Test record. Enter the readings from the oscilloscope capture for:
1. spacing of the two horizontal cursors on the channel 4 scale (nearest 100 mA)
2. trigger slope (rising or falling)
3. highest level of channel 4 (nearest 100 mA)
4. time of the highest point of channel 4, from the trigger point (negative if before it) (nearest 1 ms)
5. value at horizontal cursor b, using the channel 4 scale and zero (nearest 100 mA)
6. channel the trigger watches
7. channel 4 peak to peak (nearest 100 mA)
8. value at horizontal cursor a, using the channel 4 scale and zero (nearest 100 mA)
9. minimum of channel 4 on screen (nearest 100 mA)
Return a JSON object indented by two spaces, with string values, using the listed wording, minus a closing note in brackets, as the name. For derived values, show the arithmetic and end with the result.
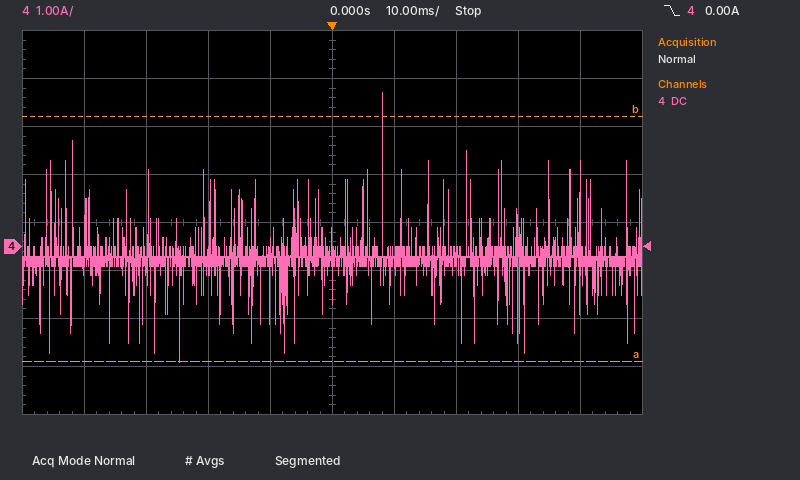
{
  "spacing of the two horizontal cursors on the channel 4 scale": "5.1 A",
  "trigger slope": "falling",
  "highest level of channel 4": "3.2 A",
  "time of the highest point of channel 4, from the trigger point (negative if before it)": "+8 ms",
  "value at horizontal cursor b, using the channel 4 scale and zero": "2.7 A",
  "channel the trigger watches": "channel 4",
  "channel 4 peak to peak": "3.2 A − (-2.4 A) = 5.6 A",
  "value at horizontal cursor a, using the channel 4 scale and zero": "-2.4 A",
  "minimum of channel 4 on screen": "-2.4 A"
}
